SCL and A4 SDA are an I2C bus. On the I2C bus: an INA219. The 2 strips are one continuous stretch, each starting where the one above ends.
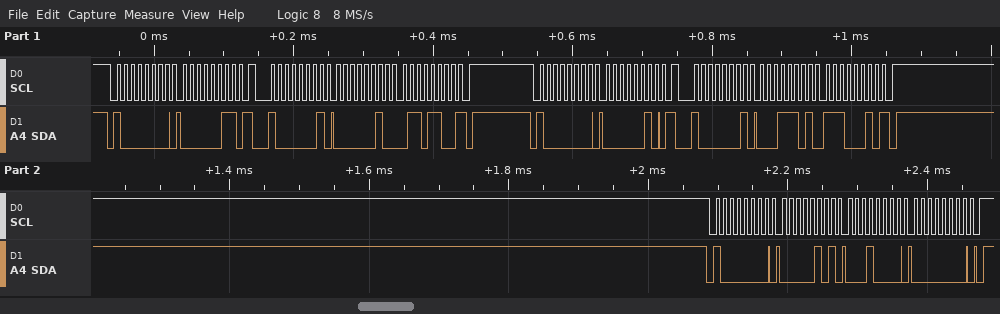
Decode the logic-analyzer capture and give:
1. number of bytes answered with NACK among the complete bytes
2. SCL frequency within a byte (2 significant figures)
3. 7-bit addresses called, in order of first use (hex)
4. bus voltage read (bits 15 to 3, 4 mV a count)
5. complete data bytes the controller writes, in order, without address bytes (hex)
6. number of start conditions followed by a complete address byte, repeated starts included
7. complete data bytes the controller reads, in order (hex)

2
100 kHz
0x40
3.824 V
03 02 05 10 00
5
02 6C 1D E2
